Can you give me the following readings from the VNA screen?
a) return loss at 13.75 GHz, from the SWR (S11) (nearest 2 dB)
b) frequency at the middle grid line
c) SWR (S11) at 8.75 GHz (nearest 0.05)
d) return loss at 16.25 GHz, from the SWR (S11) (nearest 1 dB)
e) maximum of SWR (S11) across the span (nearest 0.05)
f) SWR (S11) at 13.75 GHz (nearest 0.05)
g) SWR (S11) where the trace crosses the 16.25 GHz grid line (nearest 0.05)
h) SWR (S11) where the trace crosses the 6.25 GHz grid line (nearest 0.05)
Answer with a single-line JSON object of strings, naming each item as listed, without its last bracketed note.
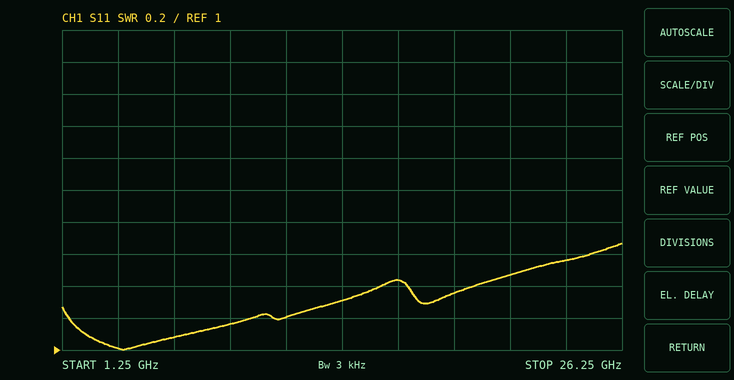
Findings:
{"return loss at 13.75 GHz, from the SWR (S11)": "18 dB", "frequency at the middle grid line": "13.75 GHz", "SWR (S11) at 8.75 GHz": "1.15", "return loss at 16.25 GHz, from the SWR (S11)": "15 dB", "maximum of SWR (S11) across the span": "1.65", "SWR (S11) at 13.75 GHz": "1.30", "SWR (S11) where the trace crosses the 16.25 GHz grid line": "1.45", "SWR (S11) where the trace crosses the 6.25 GHz grid line": "1.10"}
